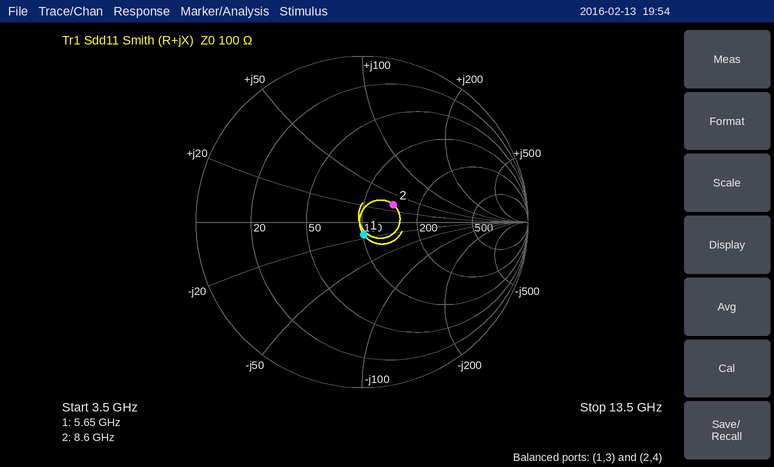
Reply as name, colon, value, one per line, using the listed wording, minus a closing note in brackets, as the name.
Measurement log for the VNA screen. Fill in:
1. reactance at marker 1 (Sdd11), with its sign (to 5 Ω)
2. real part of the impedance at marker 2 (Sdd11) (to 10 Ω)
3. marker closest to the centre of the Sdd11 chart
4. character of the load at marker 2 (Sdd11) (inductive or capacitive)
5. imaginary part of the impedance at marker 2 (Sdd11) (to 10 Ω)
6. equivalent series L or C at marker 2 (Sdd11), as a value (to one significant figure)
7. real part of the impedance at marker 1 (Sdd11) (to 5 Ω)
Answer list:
reactance at marker 1 (Sdd11), with its sign: -15 Ω
real part of the impedance at marker 2 (Sdd11): 140 Ω
marker closest to the centre of the Sdd11 chart: marker 1
character of the load at marker 2 (Sdd11): inductive
imaginary part of the impedance at marker 2 (Sdd11): +30 Ω
equivalent series L or C at marker 2 (Sdd11), as a value: 600 pH
real part of the impedance at marker 1 (Sdd11): 100 Ω
